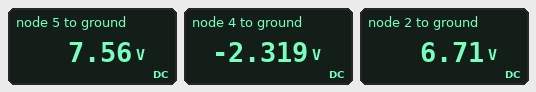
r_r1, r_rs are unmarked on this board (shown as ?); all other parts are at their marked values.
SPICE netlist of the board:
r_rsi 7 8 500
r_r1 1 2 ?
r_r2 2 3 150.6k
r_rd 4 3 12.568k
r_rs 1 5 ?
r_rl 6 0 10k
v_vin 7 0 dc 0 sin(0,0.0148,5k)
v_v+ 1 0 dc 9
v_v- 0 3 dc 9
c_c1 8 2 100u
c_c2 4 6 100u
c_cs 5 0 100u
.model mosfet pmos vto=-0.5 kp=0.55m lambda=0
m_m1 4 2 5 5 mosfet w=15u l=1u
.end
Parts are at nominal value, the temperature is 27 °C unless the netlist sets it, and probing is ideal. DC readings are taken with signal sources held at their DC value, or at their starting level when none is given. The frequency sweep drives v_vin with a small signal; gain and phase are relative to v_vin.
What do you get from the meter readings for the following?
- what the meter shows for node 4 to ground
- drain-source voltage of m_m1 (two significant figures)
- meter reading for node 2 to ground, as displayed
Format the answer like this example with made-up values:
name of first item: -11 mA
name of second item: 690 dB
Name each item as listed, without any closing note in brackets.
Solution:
what the meter shows for node 4 to ground: -2.319 V
drain-source voltage of m_m1: -9.9 V
meter reading for node 2 to ground, as displayed: 6.71 V
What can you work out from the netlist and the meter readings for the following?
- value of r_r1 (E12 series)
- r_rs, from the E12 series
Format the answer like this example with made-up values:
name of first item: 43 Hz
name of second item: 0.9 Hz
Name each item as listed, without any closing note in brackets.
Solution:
value of r_r1: 22 kΩ
r_rs, from the E12 series: 2.7 kΩ
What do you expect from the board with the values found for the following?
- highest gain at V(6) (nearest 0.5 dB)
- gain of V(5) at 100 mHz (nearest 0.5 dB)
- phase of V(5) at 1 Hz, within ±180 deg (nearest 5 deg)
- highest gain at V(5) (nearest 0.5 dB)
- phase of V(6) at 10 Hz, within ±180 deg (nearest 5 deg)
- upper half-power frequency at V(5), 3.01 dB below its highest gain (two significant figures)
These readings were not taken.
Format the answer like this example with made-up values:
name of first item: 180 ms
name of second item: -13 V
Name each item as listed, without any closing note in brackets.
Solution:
highest gain at V(6): 24.0 dB
gain of V(5) at 100 mHz: -3.5 dB
phase of V(5) at 1 Hz, within ±180 deg: -5 deg
highest gain at V(5): -1.5 dB
phase of V(6) at 10 Hz, within ±180 deg: -155 deg
upper half-power frequency at V(5), 3.01 dB below its highest gain: 5.5 Hz
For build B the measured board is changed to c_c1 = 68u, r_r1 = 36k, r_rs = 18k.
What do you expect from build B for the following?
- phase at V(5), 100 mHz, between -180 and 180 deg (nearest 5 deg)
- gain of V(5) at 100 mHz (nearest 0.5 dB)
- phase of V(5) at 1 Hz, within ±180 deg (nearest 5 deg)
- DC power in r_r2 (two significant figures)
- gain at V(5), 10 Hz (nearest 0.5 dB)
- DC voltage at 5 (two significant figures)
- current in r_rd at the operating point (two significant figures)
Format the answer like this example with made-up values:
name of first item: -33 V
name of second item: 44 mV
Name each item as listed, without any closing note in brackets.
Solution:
phase at V(5), 100 mHz, between -180 and 180 deg: 35 deg
gain of V(5) at 100 mHz: -2.5 dB
phase of V(5) at 1 Hz, within ±180 deg: -15 deg
DC power in r_r2: 1.4 mW
gain at V(5), 10 Hz: -12.5 dB
DC voltage at 5: 6.2 V
current in r_rd at the operating point: 150 µA
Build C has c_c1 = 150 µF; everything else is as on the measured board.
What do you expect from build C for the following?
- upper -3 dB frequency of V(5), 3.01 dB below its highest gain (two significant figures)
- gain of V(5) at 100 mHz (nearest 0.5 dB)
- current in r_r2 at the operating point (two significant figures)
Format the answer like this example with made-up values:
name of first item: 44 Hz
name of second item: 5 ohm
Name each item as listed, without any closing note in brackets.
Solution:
upper -3 dB frequency of V(5), 3.01 dB below its highest gain: 5.4 Hz
gain of V(5) at 100 mHz: -2.5 dB
current in r_r2 at the operating point: 100 µA
